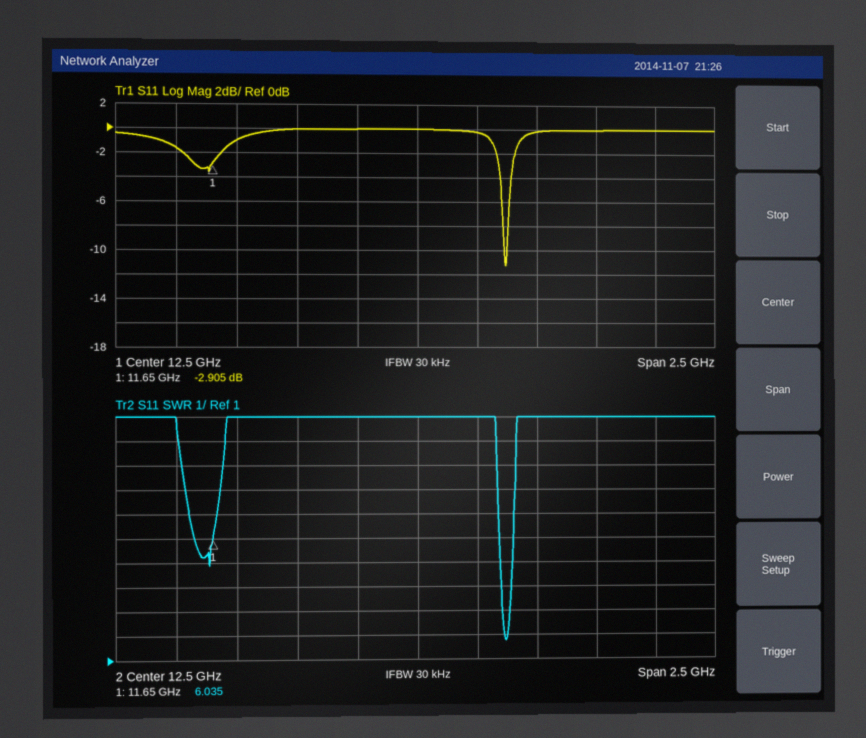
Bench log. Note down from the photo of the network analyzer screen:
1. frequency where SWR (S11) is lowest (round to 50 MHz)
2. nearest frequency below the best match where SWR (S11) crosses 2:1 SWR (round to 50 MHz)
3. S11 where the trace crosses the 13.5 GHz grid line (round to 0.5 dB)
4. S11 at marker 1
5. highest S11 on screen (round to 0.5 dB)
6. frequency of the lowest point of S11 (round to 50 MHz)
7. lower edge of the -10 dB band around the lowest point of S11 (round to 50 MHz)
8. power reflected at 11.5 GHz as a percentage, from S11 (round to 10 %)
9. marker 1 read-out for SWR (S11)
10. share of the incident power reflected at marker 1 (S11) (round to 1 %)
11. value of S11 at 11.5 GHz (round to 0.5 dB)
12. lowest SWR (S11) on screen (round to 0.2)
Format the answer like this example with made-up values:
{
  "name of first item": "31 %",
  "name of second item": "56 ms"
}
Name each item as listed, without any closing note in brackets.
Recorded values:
{
  "frequency where SWR (S11) is lowest": "12.85 GHz",
  "nearest frequency below the best match where SWR (S11) crosses 2:1 SWR": "12.85 GHz",
  "S11 where the trace crosses the 13.5 GHz grid line": "0.0 dB",
  "S11 at marker 1": "-2.905 dB",
  "highest S11 on screen": "0.0 dB",
  "frequency of the lowest point of S11": "12.85 GHz",
  "lower edge of the -10 dB band around the lowest point of S11": "12.85 GHz",
  "power reflected at 11.5 GHz as a percentage, from S11": "70 %",
  "marker 1 read-out for SWR": "6.035",
  "share of the incident power reflected at marker 1 (S11)": "51 %",
  "value of S11 at 11.5 GHz": "-1.5 dB",
  "lowest SWR (S11) on screen": "1.8"
}
